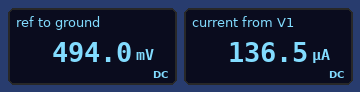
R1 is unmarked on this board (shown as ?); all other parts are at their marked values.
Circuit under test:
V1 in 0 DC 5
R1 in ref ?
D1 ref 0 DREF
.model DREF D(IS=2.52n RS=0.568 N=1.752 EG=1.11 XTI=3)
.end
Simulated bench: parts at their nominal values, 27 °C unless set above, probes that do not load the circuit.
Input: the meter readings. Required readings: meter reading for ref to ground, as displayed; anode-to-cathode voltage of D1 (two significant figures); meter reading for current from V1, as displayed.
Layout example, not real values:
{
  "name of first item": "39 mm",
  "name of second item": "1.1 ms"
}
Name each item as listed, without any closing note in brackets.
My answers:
{
  "meter reading for ref to ground, as displayed": "494.0 mV",
  "anode-to-cathode voltage of D1": "490 mV",
  "meter reading for current from V1, as displayed": "136.5 µA"
}
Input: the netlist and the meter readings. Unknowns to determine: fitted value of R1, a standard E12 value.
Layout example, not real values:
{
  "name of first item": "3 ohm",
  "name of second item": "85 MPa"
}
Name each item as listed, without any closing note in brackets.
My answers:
{
  "fitted value of R1, a standard E12 value": "33 kΩ"
}
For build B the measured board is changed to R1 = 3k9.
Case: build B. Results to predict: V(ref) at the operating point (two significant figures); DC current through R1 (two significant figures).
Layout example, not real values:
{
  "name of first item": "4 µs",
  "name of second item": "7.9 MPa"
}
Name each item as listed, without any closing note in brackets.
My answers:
{
  "V(ref) at the operating point": "590 mV",
  "DC current through R1": "1.1 mA"
}
